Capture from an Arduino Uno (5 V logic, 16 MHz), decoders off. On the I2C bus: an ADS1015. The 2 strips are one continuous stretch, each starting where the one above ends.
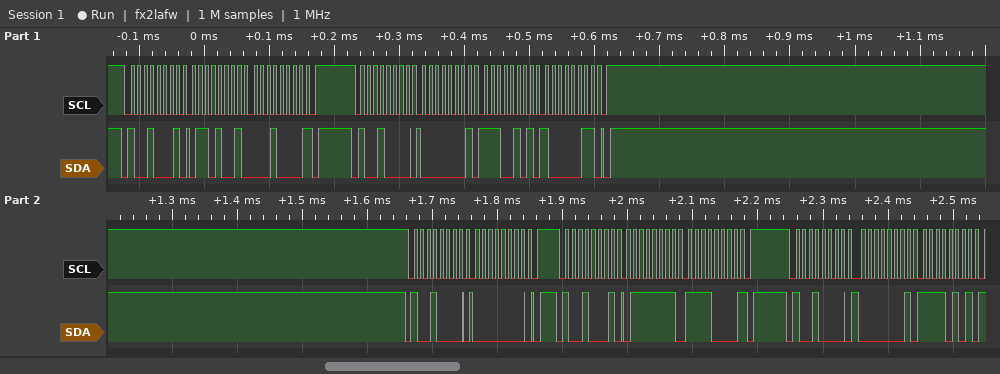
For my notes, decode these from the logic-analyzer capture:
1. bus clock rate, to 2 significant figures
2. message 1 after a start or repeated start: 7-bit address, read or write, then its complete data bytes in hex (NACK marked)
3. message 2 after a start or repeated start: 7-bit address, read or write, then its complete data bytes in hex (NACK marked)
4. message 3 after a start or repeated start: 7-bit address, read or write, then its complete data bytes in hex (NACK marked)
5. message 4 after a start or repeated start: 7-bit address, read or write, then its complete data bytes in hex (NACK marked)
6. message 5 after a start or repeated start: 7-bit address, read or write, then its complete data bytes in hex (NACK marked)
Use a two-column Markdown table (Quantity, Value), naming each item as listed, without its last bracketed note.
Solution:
| Quantity | Value |
|---|---|
| bus clock rate, to 2 significant figures | 100 kHz |
| message 1 after a start or repeated start: 7-bit address, read or write, then its complete data bytes in hex | 0x48 read: 69 10 NACK |
| message 2 after a start or repeated start: 7-bit address, read or write, then its complete data bytes in hex | 0x48 write: 01 E5 83 |
| message 3 after a start or repeated start: 7-bit address, read or write, then its complete data bytes in hex | 0x48 write: 00 |
| message 4 after a start or repeated start: 7-bit address, read or write, then its complete data bytes in hex | 0x48 read: 7F F0 NACK |
| message 5 after a start or repeated start: 7-bit address, read or write, then its complete data bytes in hex | 0x48 write: 01 F5 |
